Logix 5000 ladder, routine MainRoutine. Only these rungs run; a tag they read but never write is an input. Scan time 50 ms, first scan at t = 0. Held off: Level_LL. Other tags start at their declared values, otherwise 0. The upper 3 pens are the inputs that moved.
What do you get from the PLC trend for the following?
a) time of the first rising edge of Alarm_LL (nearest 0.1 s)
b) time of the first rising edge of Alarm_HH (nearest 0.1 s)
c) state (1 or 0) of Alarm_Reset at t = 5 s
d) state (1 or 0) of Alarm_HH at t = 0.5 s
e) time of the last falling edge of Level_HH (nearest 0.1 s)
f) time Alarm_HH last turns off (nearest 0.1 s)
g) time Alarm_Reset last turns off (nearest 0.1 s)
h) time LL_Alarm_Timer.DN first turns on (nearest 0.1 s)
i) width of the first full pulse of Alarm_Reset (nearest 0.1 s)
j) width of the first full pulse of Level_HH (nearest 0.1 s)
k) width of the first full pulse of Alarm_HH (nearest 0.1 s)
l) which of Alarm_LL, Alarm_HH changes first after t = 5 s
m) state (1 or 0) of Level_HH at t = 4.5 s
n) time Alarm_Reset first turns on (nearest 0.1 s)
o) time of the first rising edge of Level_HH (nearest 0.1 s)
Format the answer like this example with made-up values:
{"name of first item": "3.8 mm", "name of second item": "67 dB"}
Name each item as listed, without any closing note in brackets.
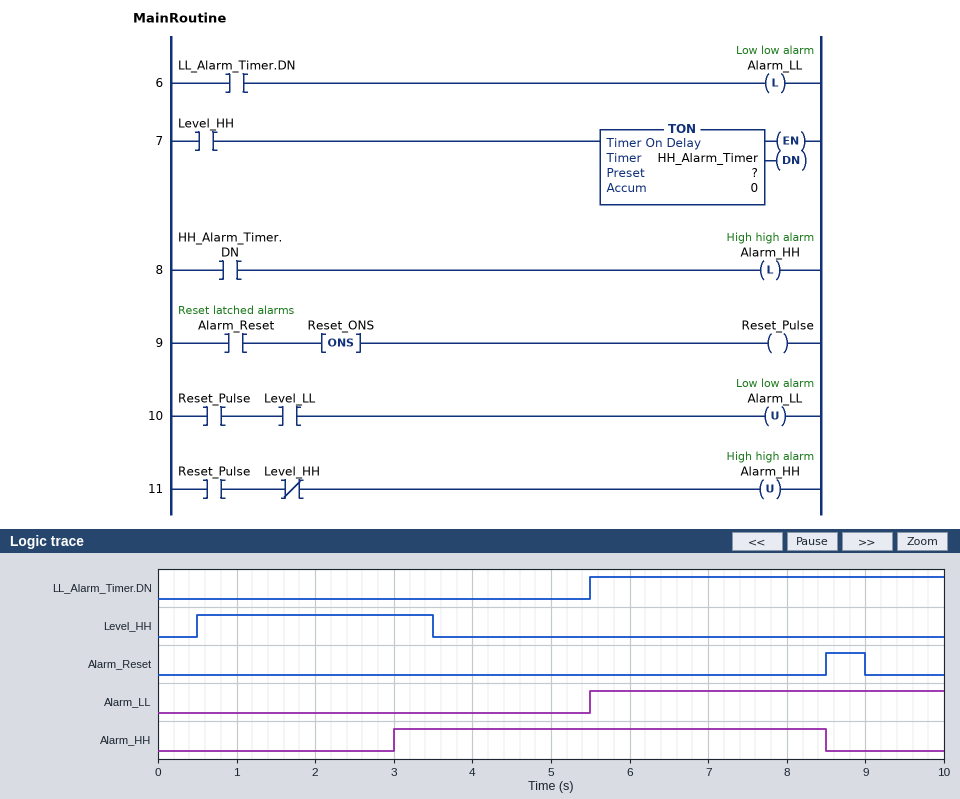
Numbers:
{"time of the first rising edge of Alarm_LL": "5.5 s", "time of the first rising edge of Alarm_HH": "3.0 s", "state (1 or 0) of Alarm_Reset at t = 5 s": "0", "state (1 or 0) of Alarm_HH at t = 0.5 s": "0", "time of the last falling edge of Level_HH": "3.5 s", "time Alarm_HH last turns off": "8.5 s", "time Alarm_Reset last turns off": "9.0 s", "time LL_Alarm_Timer.DN first turns on": "5.5 s", "width of the first full pulse of Alarm_Reset": "0.5 s", "width of the first full pulse of Level_HH": "3.0 s", "width of the first full pulse of Alarm_HH": "5.5 s", "which of Alarm_LL, Alarm_HH changes first after t = 5 s": "Alarm_LL", "state (1 or 0) of Level_HH at t = 4.5 s": "0", "time Alarm_Reset first turns on": "8.5 s", "time of the first rising edge of Level_HH": "0.5 s"}
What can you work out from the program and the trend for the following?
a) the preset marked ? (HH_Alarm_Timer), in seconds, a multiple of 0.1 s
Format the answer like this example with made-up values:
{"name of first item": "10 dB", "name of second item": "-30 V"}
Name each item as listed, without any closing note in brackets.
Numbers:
{"the preset marked ? (HH_Alarm_Timer), in seconds, a multiple of 0.1 s": "2.5 s"}
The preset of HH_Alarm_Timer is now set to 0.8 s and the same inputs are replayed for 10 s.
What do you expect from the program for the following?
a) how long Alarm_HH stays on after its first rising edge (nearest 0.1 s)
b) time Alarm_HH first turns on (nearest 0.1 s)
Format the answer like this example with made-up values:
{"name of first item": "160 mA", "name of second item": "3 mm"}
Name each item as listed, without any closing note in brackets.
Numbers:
{"how long Alarm_HH stays on after its first rising edge": "7.2 s", "time Alarm_HH first turns on": "1.3 s"}
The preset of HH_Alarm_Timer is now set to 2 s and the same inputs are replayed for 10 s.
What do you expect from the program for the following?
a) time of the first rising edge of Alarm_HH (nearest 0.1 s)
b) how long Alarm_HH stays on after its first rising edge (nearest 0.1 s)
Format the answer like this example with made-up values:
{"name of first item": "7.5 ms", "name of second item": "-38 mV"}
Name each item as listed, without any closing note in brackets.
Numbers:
{"time of the first rising edge of Alarm_HH": "2.5 s", "how long Alarm_HH stays on after its first rising edge": "6.0 s"}
